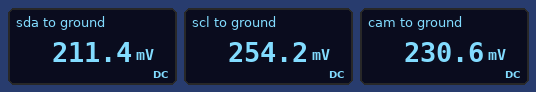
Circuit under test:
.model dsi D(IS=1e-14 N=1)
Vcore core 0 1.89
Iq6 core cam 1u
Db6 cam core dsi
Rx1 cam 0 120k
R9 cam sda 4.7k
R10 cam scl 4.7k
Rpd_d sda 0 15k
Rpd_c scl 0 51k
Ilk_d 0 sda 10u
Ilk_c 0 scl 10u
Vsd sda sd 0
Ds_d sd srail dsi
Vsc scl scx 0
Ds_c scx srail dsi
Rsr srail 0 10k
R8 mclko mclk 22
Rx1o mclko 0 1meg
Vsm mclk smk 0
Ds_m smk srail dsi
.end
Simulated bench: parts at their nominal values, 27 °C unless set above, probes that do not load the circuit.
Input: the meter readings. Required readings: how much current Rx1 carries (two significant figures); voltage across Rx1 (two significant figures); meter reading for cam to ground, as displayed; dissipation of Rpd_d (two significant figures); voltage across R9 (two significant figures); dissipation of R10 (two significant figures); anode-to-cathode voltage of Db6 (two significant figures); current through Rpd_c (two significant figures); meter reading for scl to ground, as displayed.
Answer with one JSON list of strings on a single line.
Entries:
["1.9 µA", "230 mV", "230.6 mV", "3.0 µW", "19 mV", "120 nW", "-1.7 V", "5.0 µA", "254.2 mV"]
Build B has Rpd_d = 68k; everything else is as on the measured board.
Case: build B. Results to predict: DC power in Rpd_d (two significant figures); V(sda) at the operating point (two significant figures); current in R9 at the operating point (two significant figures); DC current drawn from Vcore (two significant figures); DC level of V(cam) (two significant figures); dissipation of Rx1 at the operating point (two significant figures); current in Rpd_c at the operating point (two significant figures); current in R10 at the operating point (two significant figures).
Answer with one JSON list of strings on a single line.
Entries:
["3.3 µW", "470 mV", "2.4 µA", "1.0 µA", "460 mV", "1.8 µW", "9.1 µA", "450 nA"]
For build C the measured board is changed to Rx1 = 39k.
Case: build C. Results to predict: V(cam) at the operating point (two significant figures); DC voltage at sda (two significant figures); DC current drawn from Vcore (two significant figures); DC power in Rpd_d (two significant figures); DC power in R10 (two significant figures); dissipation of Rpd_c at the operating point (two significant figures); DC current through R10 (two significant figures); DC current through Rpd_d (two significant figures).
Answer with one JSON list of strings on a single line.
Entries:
["190 mV", "180 mV", "1.0 µA", "2.1 µW", "160 nW", "910 nW", "5.8 µA", "12 µA"]
